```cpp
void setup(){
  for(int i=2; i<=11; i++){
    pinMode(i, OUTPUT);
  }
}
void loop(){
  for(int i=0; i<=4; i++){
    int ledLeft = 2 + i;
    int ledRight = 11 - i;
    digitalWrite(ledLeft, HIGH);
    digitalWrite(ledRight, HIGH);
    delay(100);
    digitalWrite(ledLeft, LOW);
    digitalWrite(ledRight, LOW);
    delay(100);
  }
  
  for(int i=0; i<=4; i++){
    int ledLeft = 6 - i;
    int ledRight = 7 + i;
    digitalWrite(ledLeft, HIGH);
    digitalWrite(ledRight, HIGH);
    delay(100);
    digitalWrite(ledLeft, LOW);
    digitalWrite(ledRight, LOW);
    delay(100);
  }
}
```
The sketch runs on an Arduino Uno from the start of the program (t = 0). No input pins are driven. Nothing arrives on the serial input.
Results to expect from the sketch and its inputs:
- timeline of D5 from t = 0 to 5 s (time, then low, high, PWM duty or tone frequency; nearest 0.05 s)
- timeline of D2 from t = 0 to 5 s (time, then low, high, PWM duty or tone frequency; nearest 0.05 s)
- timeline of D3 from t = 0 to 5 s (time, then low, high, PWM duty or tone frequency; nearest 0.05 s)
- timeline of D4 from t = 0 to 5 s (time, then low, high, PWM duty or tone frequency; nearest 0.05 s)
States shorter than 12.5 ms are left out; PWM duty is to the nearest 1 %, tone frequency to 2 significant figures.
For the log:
0 s low; 0.6 s high; 0.7 s low; 1.2 s high; 1.3 s low; 2.6 s high; 2.7 s low; 3.2 s high; 3.3 s low; 4.6 s high; 4.7 s low
0 s high; 0.1 s low; 1.8 s high; 1.9 s low; 2 s high; 2.1 s low; 3.8 s high; 3.9 s low; 4 s high; 4.1 s low
0 s low; 0.2 s high; 0.3 s low; 1.6 s high; 1.7 s low; 2.2 s high; 2.3 s low; 3.6 s high; 3.7 s low; 4.2 s high; 4.3 s low
0 s low; 0.4 s high; 0.5 s low; 1.4 s high; 1.5 s low; 2.4 s high; 2.5 s low; 3.4 s high; 3.5 s low; 4.4 s high; 4.5 s low
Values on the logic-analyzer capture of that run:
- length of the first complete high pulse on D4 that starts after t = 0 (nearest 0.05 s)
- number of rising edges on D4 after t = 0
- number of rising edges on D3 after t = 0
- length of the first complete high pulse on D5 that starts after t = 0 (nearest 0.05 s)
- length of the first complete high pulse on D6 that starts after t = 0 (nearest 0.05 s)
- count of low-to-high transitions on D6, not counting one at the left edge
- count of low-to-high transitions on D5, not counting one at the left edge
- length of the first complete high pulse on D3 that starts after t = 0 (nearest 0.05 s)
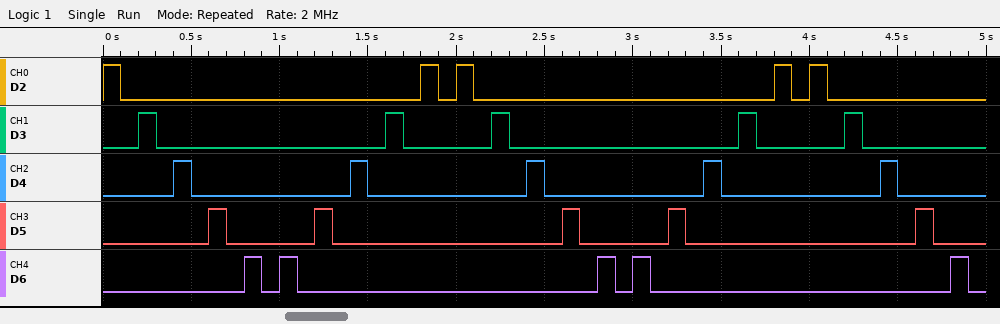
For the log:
0.10 s
5
5
0.10 s
0.10 s
5
5
0.10 s
